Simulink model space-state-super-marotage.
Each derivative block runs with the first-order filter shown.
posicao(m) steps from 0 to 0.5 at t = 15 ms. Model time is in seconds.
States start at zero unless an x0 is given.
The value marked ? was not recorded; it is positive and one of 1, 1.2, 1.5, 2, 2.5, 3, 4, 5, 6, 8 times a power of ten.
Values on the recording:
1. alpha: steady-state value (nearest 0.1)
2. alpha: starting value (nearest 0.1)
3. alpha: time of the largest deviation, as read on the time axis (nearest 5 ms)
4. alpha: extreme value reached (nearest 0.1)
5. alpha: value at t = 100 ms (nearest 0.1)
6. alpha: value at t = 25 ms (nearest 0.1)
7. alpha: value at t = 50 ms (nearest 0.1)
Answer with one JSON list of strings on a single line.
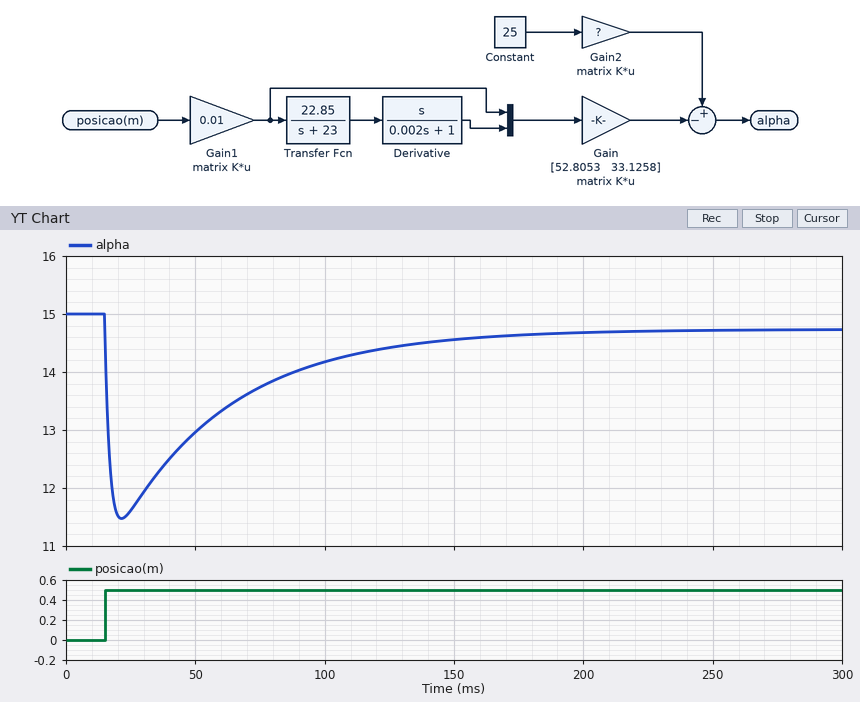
["14.7", "15.0", "20 ms", "11.5", "14.2", "11.6", "13.0"]
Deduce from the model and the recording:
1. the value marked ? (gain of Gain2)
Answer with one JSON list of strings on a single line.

["0.6"]
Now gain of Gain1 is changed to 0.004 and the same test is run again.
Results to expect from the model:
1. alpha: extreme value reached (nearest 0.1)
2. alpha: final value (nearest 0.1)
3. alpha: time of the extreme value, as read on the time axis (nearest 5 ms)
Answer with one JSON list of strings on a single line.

["13.6", "14.9", "20 ms"]
